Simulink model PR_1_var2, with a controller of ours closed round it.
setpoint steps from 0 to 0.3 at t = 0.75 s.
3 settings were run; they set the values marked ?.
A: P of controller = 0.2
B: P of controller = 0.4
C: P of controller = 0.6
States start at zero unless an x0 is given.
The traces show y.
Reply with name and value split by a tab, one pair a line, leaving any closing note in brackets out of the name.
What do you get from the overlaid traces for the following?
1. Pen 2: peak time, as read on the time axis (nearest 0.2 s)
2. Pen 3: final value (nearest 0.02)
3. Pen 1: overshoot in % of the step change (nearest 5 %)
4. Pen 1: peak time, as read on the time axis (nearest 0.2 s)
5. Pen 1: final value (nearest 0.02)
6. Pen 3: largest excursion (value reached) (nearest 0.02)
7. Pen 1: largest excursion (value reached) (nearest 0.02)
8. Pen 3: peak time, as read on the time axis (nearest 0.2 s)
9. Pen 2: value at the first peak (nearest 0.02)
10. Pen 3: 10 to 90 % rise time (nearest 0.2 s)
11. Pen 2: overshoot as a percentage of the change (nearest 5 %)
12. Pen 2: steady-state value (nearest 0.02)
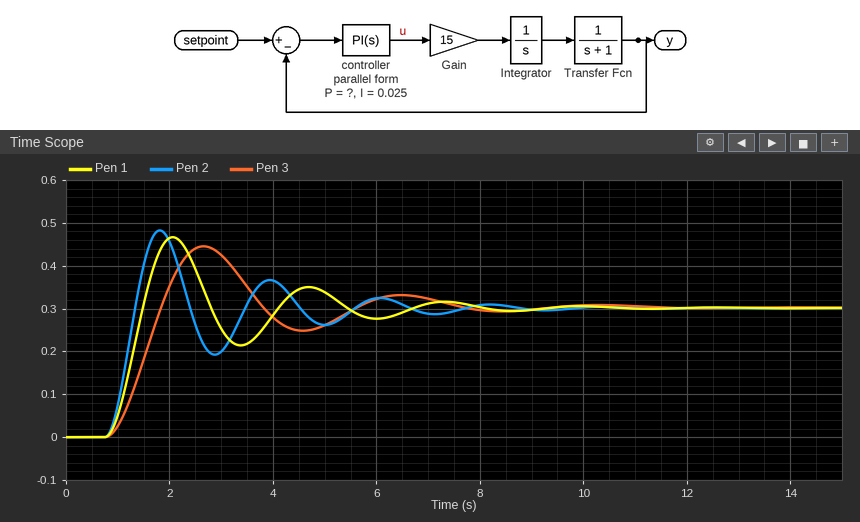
Pen 2: peak time, as read on the time axis	1.8 s
Pen 3: final value	0.30
Pen 1: overshoot in % of the step change	55 %
Pen 1: peak time, as read on the time axis	2.0 s
Pen 1: final value	0.30
Pen 3: largest excursion (value reached)	0.44
Pen 1: largest excursion (value reached)	0.46
Pen 3: peak time, as read on the time axis	2.6 s
Pen 2: value at the first peak	0.48
Pen 3: 10 to 90 % rise time	0.8 s
Pen 2: overshoot as a percentage of the change	60 %
Pen 2: steady-state value	0.30
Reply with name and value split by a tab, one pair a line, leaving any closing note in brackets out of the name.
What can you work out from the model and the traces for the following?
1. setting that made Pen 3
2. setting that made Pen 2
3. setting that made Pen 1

setting that made Pen 3	A
setting that made Pen 2	C
setting that made Pen 1	B
